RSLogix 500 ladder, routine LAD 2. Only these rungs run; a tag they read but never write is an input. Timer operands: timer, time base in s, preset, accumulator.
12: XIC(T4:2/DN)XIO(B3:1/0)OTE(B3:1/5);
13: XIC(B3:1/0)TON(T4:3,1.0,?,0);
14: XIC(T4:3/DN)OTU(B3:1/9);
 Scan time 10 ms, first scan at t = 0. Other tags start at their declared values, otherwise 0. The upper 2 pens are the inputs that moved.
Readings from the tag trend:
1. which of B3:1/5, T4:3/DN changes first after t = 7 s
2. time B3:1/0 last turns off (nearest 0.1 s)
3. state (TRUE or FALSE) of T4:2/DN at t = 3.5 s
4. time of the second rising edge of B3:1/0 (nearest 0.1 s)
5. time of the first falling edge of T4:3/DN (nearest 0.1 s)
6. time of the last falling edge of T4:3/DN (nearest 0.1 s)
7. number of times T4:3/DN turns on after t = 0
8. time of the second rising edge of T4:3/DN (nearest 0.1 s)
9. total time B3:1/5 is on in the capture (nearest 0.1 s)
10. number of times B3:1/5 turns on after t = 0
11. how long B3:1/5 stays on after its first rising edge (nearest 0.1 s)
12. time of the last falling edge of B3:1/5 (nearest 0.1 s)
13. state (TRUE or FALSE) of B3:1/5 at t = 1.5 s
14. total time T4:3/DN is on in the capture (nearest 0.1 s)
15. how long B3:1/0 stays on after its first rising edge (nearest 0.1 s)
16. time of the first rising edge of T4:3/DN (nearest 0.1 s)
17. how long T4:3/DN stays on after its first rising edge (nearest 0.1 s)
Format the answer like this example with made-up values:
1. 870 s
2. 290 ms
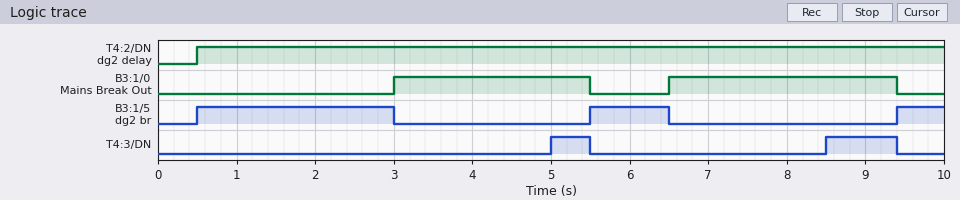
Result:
1. T4:3/DN
2. 9.4 s
3. TRUE
4. 6.5 s
5. 5.5 s
6. 9.4 s
7. 2
8. 8.5 s
9. 4.1 s
10. 3
11. 2.5 s
12. 6.5 s
13. TRUE
14. 1.4 s
15. 2.5 s
16. 5.0 s
17. 0.5 s
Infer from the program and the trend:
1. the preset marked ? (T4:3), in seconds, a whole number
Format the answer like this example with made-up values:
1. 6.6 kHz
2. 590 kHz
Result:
1. 2 s
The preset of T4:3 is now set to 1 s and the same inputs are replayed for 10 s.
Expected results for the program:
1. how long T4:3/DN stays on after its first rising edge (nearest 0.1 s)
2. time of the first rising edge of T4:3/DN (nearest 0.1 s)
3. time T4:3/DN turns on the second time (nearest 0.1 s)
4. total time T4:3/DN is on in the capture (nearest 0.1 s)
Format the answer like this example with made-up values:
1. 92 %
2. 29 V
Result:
1. 1.5 s
2. 4.0 s
3. 7.5 s
4. 3.4 s
